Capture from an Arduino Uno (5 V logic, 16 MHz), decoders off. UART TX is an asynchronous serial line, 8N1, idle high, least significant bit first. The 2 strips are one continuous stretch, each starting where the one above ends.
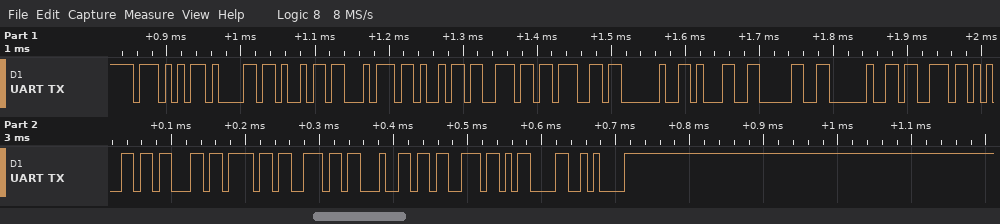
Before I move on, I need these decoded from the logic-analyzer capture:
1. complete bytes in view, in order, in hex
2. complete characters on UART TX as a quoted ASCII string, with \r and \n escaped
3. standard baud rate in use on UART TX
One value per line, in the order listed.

57 61 69 74 69 6E 67 20 31 30 20 73 65 63 6F 6E 64 73 0D 0A
"Waiting 10 seconds\r\n"
115200 baud
